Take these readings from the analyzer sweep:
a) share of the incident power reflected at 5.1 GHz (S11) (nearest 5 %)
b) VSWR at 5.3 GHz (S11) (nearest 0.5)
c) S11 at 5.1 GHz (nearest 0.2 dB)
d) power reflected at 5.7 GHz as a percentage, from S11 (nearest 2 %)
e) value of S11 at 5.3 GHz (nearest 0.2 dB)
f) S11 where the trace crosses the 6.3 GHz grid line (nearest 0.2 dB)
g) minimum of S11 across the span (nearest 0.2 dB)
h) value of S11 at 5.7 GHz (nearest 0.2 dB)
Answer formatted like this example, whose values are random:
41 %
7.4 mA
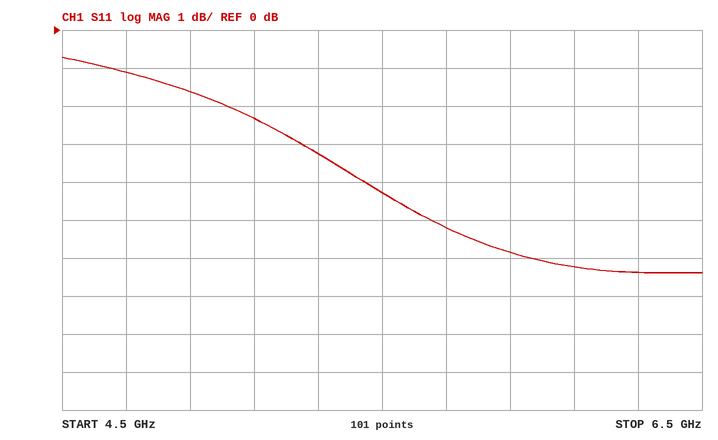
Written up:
60 %
5.5
-2.4 dB
30 %
-3.2 dB
-6.4 dB
-6.4 dB
-5.2 dB
